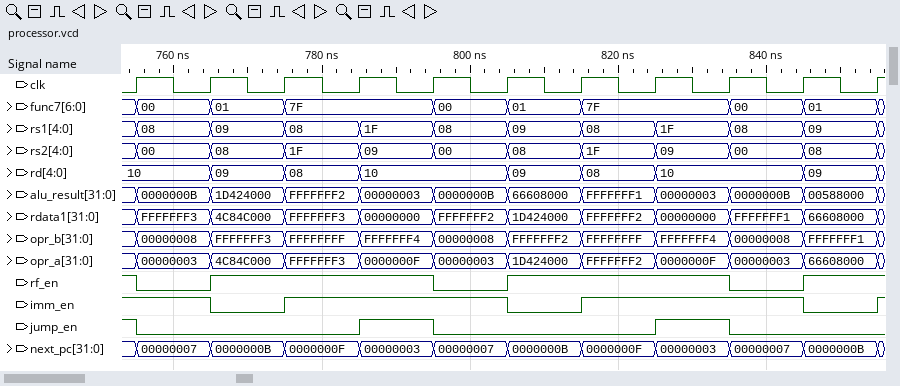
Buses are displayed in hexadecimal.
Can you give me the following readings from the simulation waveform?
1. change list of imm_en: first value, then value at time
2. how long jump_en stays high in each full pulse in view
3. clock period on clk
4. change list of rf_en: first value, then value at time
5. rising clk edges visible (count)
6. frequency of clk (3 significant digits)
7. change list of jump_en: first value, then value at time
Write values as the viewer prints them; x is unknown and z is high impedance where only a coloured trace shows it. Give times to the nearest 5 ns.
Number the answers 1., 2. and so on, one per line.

1. 1, 0 at 765 ns, 1 at 775 ns, 0 at 805 ns, 1 at 815 ns, 0 at 845 ns, 1 at 855 ns
2. 10 ns, 10 ns
3. 10 ns
4. 1, 0 at 755 ns, 1 at 765 ns, 0 at 795 ns, 1 at 805 ns, 0 at 835 ns, 1 at 845 ns
5. 11
6. 100 MHz
7. 1, 0 at 755 ns, 1 at 785 ns, 0 at 795 ns, 1 at 825 ns, 0 at 835 ns
